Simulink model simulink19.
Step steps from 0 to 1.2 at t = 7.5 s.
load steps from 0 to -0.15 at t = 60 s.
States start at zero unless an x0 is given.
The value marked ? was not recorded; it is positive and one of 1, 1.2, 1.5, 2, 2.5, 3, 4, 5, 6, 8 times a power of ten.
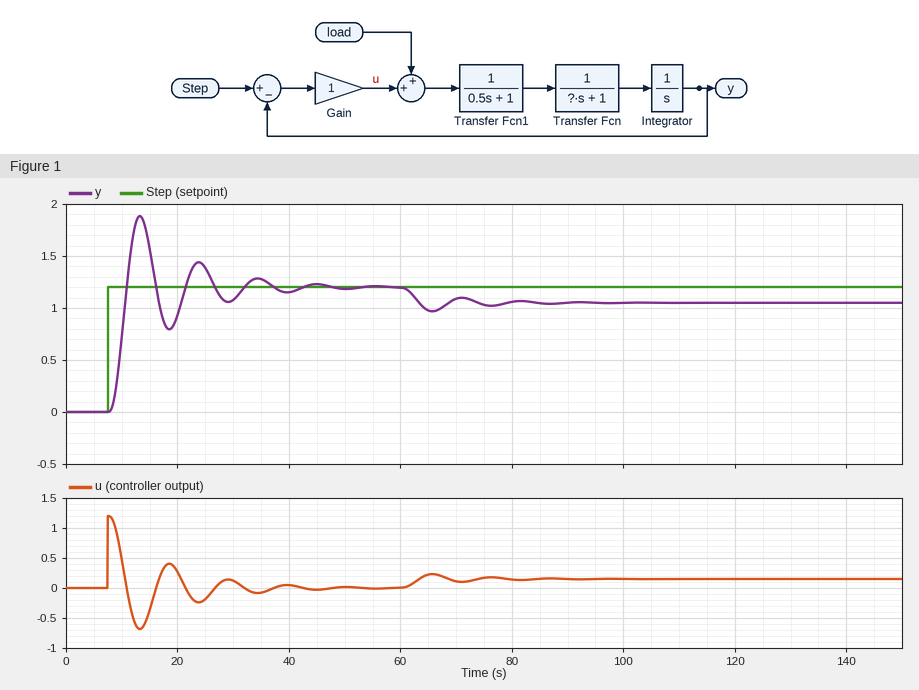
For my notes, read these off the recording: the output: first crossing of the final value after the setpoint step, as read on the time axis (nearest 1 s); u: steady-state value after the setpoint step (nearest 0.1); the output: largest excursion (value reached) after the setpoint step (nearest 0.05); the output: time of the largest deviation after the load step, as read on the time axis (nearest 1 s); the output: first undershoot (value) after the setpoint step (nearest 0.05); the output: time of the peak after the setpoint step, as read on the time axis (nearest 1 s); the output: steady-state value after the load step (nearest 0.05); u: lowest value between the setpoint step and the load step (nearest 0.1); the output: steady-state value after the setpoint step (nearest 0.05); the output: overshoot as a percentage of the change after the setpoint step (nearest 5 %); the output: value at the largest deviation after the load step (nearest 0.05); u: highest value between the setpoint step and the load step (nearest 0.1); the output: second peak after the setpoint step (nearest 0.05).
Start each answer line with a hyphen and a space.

- 11 s
- 0.0
- 1.90
- 66 s
- 0.80
- 13 s
- 1.05
- -0.7
- 1.20
- 55 %
- 0.95
- 1.2
- 1.45
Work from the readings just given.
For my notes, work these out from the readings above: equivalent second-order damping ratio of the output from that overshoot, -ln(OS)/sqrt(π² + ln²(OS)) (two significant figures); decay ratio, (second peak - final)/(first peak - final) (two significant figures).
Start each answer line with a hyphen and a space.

- 0.19
- 0.36
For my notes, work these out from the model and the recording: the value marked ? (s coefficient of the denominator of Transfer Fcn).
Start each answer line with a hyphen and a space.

- 2.5
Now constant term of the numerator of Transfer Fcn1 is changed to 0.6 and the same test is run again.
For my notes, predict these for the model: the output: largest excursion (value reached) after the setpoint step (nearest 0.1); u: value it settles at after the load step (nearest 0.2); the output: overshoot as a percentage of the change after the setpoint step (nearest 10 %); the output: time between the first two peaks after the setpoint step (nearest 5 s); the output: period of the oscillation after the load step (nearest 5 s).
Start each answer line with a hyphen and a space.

- 1.7
- 0.2
- 40 %
- 15 s
- 15 s
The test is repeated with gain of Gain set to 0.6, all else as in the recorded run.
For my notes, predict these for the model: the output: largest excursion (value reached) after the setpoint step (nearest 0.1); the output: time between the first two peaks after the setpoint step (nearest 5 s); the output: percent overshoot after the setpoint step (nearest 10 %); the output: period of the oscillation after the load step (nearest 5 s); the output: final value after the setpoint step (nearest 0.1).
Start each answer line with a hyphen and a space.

- 1.7
- 15 s
- 40 %
- 15 s
- 1.2
